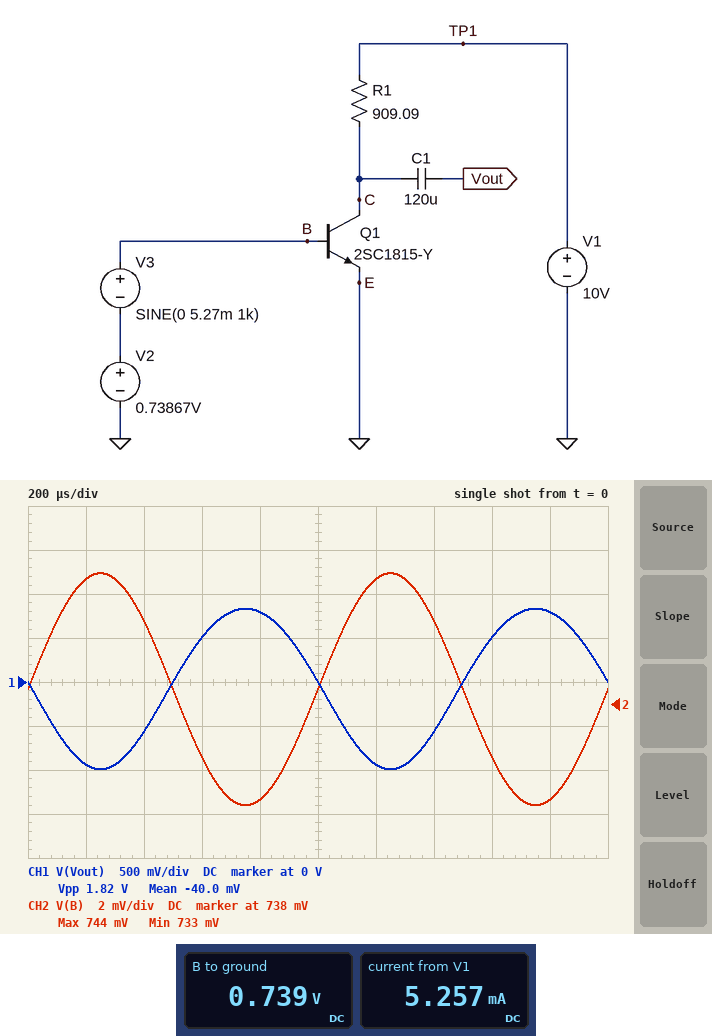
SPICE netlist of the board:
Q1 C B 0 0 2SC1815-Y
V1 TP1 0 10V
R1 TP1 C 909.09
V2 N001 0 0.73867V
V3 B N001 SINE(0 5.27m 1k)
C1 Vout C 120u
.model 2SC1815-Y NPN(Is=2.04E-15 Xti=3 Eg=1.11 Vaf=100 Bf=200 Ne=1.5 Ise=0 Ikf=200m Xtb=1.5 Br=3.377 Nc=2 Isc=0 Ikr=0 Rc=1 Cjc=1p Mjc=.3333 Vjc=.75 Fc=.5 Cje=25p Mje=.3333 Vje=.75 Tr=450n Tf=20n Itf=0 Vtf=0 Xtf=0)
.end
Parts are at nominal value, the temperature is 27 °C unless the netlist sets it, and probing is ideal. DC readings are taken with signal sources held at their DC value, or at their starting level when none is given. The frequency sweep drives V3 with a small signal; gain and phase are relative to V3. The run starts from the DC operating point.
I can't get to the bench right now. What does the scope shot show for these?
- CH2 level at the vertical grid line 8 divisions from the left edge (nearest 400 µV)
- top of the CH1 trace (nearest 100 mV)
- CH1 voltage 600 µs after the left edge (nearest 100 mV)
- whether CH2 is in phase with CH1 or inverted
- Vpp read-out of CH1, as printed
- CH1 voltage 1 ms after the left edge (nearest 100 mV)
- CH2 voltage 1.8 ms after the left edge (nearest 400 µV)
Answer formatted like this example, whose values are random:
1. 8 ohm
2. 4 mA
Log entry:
1. 735.6 mV
2. 800 mV
3. 500 mV
4. inverted
5. 1.82 V
6. 0 V
7. 733.6 mV
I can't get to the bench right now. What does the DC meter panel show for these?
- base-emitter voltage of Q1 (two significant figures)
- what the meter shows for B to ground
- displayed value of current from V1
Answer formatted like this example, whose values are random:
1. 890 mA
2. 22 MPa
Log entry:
1. 740 mV
2. 0.739 V
3. 5.257 mA
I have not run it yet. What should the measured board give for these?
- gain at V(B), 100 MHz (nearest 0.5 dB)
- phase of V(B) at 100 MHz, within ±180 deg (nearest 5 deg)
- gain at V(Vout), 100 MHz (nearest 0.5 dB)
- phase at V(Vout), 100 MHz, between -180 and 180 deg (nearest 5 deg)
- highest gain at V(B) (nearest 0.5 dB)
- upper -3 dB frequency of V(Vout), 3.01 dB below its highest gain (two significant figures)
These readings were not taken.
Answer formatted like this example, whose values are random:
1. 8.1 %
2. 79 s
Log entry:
1. 0 dB
2. 0 deg
3. 44.5 dB
4. 165 deg
5. 0 dB
6. 350 MHz
